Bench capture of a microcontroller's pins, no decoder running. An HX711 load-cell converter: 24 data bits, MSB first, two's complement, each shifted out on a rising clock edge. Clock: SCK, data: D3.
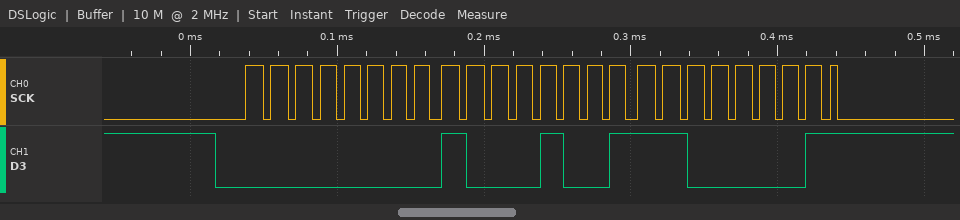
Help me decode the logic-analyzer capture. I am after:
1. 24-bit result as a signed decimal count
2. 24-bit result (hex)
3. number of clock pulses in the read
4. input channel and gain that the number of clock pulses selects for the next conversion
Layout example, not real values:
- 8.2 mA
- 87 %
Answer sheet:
- 35265
- 0x0089C1
- 25
- channel A, gain 128
